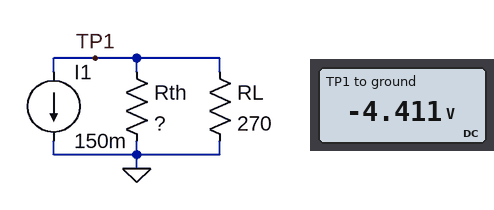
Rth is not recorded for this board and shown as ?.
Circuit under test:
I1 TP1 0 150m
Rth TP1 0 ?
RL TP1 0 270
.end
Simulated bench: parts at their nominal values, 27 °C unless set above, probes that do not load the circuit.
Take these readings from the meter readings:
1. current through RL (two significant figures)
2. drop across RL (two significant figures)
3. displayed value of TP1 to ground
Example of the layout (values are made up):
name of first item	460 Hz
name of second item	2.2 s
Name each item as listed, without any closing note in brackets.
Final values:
current through RL	16 mA
drop across RL	4.4 V
displayed value of TP1 to ground	-4.411 V
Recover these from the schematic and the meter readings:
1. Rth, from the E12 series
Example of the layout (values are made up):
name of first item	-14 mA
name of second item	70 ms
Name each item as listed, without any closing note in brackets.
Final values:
Rth, from the E12 series	33 Ω
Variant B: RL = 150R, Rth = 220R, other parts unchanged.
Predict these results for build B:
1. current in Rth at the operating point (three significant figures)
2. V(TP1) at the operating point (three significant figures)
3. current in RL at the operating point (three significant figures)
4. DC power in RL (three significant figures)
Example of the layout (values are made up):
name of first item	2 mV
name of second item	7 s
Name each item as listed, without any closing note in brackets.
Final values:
current in Rth at the operating point	60.8 mA
V(TP1) at the operating point	-13.4 V
current in RL at the operating point	89.2 mA
DC power in RL	1.19 W
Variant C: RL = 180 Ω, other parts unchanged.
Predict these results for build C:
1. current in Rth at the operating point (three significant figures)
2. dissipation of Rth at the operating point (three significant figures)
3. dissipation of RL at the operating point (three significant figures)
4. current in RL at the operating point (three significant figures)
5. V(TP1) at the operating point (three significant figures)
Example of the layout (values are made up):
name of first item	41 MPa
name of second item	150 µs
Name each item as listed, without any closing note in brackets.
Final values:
current in Rth at the operating point	127 mA
dissipation of Rth at the operating point	530 mW
dissipation of RL at the operating point	97.2 mW
current in RL at the operating point	23.2 mA
V(TP1) at the operating point	-4.18 V
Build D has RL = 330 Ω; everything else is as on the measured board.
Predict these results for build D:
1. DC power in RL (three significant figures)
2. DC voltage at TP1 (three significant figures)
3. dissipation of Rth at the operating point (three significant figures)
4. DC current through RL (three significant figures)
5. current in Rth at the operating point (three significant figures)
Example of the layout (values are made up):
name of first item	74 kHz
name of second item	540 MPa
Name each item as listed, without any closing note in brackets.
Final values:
DC power in RL	61.4 mW
DC voltage at TP1	-4.50 V
dissipation of Rth at the operating point	614 mW
DC current through RL	13.6 mA
current in Rth at the operating point	136 mA
